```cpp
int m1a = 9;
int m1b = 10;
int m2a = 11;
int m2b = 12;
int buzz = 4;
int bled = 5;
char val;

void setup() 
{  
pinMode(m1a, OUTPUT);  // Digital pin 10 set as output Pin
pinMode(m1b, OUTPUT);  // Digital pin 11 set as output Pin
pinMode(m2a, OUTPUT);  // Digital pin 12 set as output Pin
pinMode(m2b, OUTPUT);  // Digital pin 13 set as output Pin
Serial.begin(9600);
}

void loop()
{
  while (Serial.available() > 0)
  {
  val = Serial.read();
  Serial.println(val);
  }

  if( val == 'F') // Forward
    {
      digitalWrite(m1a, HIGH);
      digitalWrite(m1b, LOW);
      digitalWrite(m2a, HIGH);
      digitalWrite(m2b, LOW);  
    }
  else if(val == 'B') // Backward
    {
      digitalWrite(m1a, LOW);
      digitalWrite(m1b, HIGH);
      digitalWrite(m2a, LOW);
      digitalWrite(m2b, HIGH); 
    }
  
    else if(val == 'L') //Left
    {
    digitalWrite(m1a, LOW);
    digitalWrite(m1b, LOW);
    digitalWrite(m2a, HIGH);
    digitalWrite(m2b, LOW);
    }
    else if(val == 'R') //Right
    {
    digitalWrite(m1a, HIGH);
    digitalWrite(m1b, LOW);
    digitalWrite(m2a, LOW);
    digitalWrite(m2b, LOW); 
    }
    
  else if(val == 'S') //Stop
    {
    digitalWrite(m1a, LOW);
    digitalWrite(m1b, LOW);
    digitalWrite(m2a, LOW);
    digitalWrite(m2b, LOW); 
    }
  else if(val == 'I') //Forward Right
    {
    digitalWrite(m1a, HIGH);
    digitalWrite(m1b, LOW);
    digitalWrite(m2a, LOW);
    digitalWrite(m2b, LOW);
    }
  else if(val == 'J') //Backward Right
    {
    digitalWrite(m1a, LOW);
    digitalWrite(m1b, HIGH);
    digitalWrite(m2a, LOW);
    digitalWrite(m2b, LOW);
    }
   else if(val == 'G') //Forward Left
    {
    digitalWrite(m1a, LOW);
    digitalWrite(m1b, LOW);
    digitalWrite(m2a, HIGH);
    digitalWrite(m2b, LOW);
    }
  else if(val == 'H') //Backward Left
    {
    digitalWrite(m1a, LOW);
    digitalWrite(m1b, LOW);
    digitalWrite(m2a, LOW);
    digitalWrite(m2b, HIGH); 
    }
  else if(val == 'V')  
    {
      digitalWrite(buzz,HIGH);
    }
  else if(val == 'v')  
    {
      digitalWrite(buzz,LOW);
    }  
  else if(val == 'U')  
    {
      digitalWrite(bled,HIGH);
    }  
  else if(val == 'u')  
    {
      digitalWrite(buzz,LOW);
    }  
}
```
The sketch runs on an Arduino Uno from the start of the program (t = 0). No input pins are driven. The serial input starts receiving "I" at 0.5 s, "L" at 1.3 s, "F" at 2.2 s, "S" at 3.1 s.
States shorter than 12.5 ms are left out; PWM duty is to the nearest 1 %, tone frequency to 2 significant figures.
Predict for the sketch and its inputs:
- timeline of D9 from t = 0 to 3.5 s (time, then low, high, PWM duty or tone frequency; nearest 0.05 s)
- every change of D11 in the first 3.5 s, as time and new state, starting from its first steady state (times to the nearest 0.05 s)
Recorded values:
0 s low; 0.5 s high; 1.3 s low; 2.2 s high; 3.1 s low
0 s low; 1.3 s high; 3.1 s low
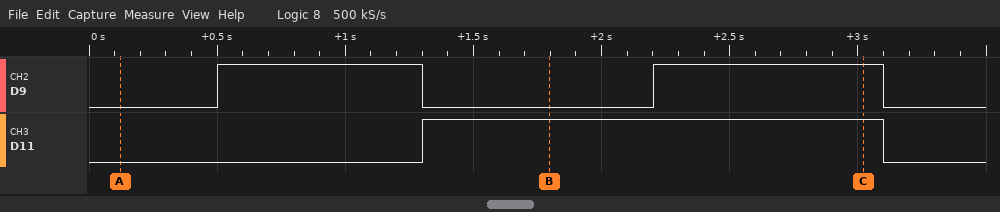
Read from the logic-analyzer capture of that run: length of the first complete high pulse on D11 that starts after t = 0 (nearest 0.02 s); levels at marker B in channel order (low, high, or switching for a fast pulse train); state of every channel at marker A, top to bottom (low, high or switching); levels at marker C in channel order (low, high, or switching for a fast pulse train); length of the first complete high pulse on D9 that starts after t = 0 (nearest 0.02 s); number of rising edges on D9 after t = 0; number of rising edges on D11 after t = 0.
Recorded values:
1.80 s
D9 low, D11 high
D9 low, D11 low
D9 high, D11 high
0.80 s
2
1
